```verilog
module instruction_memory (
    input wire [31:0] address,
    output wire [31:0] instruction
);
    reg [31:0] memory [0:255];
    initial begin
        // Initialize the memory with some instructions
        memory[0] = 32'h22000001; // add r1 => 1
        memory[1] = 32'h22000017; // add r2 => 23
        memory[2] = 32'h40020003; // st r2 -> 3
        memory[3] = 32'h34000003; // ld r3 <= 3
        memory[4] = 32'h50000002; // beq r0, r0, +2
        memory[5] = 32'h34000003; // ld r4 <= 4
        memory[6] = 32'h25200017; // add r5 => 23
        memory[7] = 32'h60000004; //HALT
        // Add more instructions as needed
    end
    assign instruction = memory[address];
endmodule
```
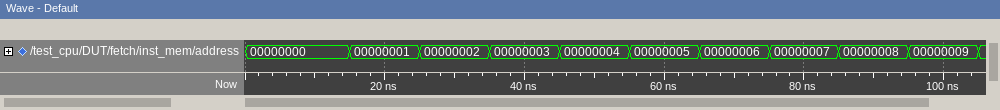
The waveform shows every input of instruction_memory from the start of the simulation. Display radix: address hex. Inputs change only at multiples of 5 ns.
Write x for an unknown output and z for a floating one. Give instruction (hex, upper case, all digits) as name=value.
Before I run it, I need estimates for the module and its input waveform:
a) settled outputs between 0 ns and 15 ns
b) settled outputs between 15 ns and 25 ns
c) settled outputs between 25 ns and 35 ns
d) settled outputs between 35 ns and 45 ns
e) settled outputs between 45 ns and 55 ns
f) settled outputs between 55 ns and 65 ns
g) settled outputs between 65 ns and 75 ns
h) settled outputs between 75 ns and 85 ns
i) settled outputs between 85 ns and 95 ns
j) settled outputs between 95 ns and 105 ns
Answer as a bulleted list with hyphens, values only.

- instruction=22000001
- instruction=22000017
- instruction=40020003
- instruction=34000003
- instruction=50000002
- instruction=34000003
- instruction=25200017
- instruction=60000004
- instruction=x
- instruction=x
